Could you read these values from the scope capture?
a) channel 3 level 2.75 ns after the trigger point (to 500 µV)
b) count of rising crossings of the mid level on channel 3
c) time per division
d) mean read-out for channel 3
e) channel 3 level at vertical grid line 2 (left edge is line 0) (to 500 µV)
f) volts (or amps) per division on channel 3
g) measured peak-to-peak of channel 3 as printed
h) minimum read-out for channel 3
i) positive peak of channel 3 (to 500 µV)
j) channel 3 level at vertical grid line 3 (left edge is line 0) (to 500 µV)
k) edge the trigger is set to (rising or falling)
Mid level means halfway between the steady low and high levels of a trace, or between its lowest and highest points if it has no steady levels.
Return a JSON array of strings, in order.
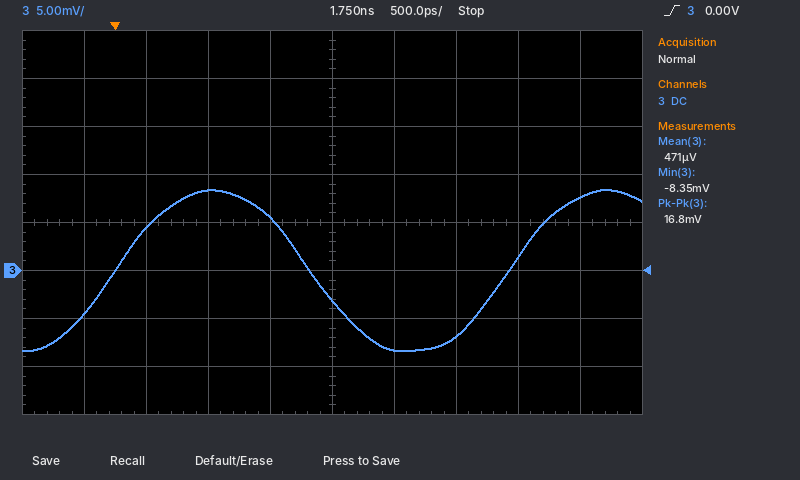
["-7.0 mV", "2", "500 ps", "471 µV", "4.5 mV", "5 mV", "16.8 mV", "-8.35 mV", "8.5 mV", "8.5 mV", "rising"]
